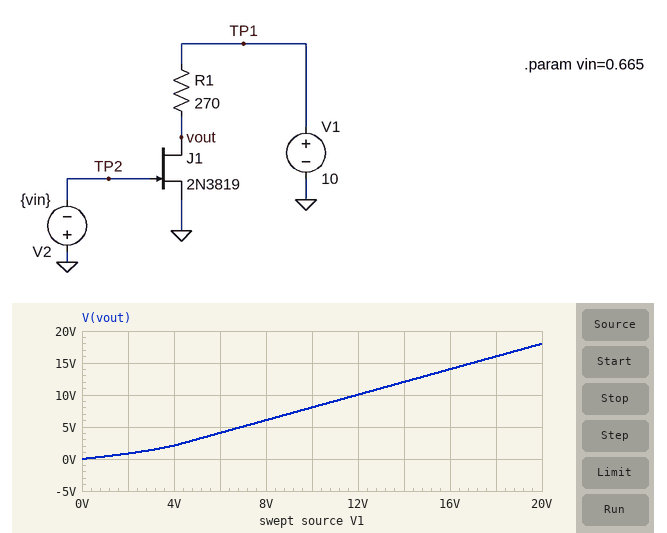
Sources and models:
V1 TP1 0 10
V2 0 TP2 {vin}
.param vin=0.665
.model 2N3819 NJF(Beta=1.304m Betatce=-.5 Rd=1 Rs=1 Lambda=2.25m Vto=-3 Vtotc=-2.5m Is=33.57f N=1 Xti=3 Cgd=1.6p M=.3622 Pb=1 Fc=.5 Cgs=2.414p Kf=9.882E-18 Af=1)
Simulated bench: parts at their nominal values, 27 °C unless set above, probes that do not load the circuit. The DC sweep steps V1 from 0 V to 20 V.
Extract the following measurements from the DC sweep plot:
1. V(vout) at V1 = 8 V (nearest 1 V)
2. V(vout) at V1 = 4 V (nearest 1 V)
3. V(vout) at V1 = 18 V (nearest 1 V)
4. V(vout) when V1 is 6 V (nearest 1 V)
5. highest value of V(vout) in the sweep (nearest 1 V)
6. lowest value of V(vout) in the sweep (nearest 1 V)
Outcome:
6 V
2 V
16 V
4 V
18 V
0 V
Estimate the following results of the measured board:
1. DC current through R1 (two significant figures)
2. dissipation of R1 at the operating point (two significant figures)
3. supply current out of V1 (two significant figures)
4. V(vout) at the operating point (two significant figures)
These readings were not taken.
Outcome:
7.2 mA
14 mW
7.2 mA
8.1 V
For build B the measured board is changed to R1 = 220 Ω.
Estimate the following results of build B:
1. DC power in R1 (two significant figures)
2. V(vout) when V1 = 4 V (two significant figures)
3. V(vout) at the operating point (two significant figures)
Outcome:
11 mW
2.4 V
8.4 V
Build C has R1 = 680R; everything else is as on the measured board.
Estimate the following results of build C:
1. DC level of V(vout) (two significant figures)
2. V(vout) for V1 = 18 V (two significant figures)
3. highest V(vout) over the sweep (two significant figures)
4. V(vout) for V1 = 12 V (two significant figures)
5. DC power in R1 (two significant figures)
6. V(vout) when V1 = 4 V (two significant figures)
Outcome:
5.1 V
13 V
15 V
7.1 V
35 mW
930 mV
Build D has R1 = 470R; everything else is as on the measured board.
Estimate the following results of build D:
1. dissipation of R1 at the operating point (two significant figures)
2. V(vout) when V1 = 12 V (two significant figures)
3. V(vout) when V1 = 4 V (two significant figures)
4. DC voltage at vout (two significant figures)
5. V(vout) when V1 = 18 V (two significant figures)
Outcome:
24 mW
8.6 V
1.3 V
6.6 V
15 V
